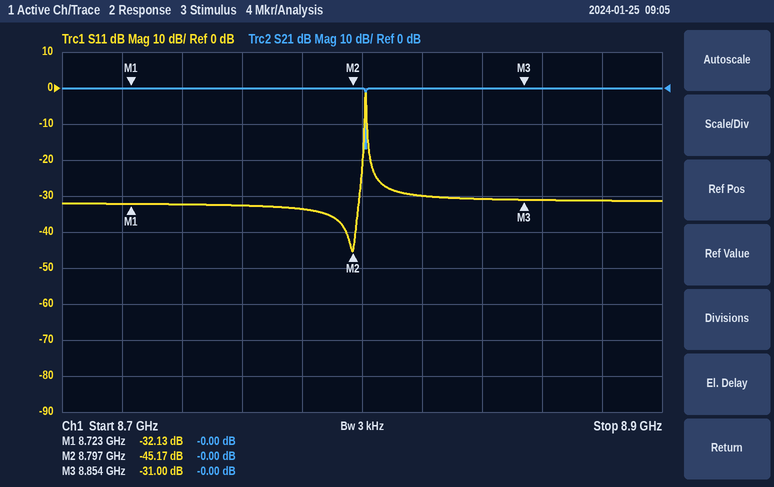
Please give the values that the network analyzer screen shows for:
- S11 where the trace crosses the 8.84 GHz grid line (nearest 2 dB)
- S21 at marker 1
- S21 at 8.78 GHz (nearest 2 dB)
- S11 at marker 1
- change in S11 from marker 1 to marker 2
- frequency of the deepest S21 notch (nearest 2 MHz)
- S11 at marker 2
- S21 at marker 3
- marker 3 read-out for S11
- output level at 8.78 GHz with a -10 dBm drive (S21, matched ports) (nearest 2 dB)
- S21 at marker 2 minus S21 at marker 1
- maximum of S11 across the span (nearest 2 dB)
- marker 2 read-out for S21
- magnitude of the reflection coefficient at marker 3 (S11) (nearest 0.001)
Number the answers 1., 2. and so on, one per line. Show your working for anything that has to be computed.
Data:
1. -30 dB
2. -0.00 dB
3. 0 dB
4. -32.13 dB
5. -45.17 − (-32.13) = -13.04 dB
6. 8.802 GHz
7. -45.17 dB
8. -0.00 dB
9. -31.00 dB
10. -10 dBm + (0 dB) = -10 dBm
11. -0 − (-0) = 0.00 dB
12. -2 dB
13. -0.00 dB
14. 10^(-31/20) ≈ 0.028
